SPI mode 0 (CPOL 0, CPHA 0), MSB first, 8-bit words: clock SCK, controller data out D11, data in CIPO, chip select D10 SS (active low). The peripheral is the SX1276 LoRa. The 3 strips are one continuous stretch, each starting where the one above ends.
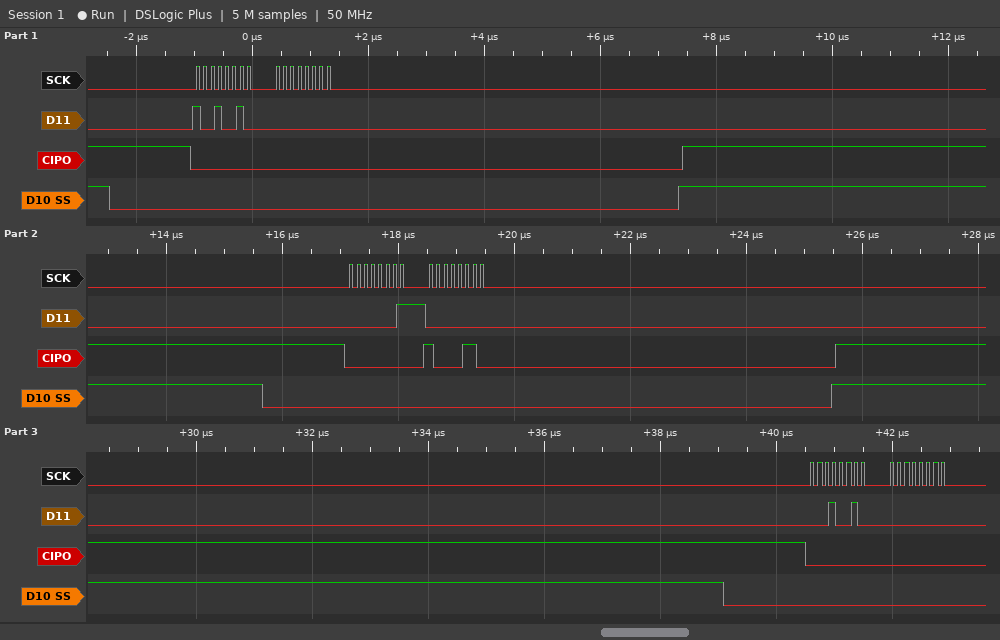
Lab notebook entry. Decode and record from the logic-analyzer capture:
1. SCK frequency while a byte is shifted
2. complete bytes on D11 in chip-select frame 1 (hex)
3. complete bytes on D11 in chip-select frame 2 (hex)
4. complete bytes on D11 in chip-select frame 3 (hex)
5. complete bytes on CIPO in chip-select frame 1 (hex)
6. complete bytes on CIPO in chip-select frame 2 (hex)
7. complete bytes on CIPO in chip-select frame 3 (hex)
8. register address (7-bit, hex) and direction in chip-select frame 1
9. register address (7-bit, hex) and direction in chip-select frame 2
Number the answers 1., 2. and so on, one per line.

1. 8 MHz
2. 92 00
3. 01 00
4. 12 00
5. 00 00
6. 00 86
7. 00 00
8. 0x12 write
9. 0x01 read
